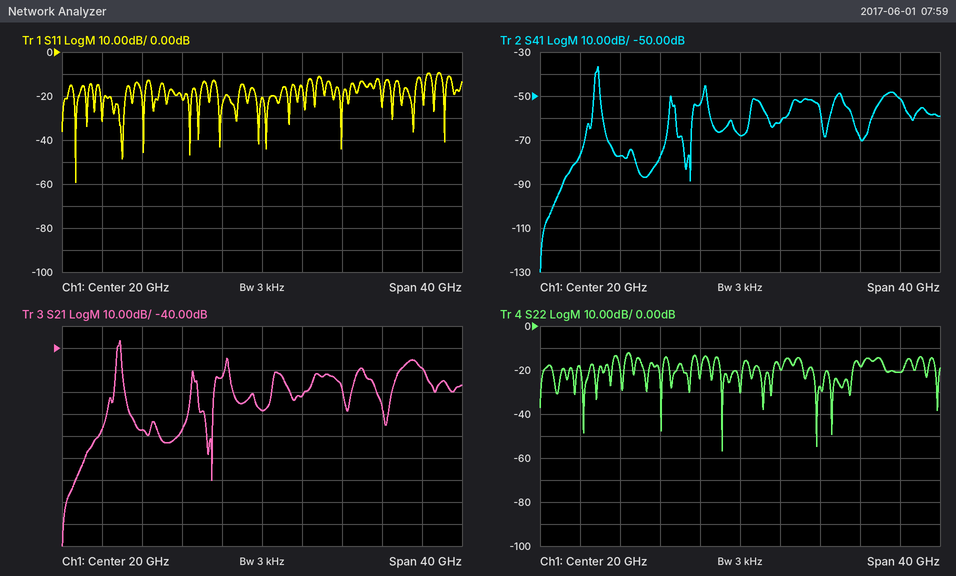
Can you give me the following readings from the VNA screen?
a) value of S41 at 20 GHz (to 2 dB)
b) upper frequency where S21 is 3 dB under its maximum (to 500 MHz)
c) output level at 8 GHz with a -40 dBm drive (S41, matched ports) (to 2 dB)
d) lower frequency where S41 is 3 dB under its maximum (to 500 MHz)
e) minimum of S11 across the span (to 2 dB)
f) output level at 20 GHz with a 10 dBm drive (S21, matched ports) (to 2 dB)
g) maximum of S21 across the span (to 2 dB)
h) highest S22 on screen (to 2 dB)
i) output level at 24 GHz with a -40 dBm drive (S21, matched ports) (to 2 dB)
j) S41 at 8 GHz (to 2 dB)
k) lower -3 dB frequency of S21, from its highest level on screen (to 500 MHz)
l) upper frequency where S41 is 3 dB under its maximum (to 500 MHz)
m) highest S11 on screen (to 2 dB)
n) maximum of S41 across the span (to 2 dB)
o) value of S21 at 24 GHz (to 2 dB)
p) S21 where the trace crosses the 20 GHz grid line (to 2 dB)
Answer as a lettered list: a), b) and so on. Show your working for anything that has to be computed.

a) -68 dB
b) 6.0 GHz
c) -40 dBm + (-78 dB) = -118 dBm
d) 5.5 GHz
e) -60 dB
f) 10 dBm + (-68 dB) = -58 dBm
g) -36 dB
h) -12 dB
i) -40 dBm + (-62 dB) = -102 dBm
j) -78 dB
k) 5.5 GHz
l) 6.0 GHz
m) -10 dB
n) -36 dB
o) -62 dB
p) -68 dB
